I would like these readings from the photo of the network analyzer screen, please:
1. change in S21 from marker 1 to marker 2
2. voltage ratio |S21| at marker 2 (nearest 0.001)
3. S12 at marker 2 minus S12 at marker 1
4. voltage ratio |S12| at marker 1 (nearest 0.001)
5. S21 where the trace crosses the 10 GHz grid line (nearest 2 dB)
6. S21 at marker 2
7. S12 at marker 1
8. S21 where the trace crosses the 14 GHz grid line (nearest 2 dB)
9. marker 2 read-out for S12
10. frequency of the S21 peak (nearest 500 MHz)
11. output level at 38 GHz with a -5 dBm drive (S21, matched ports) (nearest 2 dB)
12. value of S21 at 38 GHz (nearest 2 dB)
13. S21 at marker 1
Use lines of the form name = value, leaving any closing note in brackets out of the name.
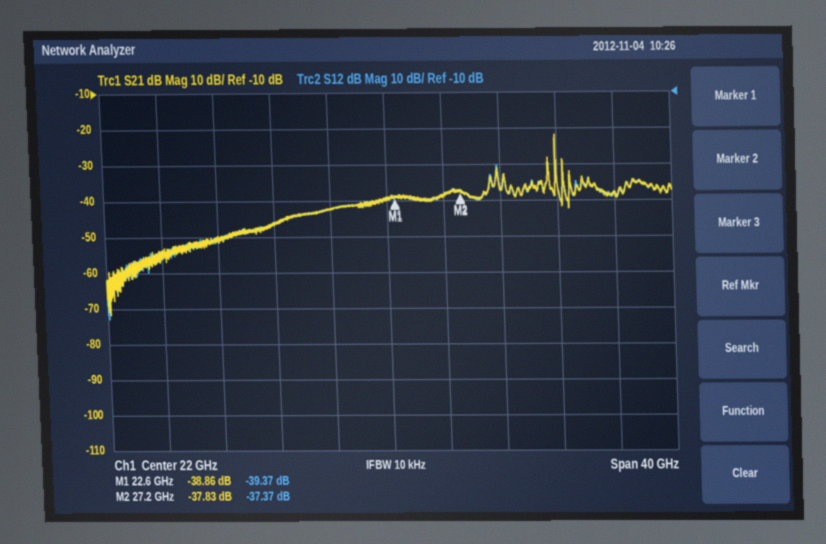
change in S21 from marker 1 to marker 2 = 1.03 dB
voltage ratio |S21| at marker 2 = 0.013
S12 at marker 2 minus S12 at marker 1 = 2.00 dB
voltage ratio |S12| at marker 1 = 0.011
S21 where the trace crosses the 10 GHz grid line = -50 dB
S21 at marker 2 = -37.83 dB
S12 at marker 1 = -39.37 dB
S21 where the trace crosses the 14 GHz grid line = -46 dB
marker 2 read-out for S12 = -37.37 dB
frequency of the S21 peak = 34.0 GHz
output level at 38 GHz with a -5 dBm drive (S21, matched ports) = -44 dBm
value of S21 at 38 GHz = -38 dB
S21 at marker 1 = -38.86 dB
